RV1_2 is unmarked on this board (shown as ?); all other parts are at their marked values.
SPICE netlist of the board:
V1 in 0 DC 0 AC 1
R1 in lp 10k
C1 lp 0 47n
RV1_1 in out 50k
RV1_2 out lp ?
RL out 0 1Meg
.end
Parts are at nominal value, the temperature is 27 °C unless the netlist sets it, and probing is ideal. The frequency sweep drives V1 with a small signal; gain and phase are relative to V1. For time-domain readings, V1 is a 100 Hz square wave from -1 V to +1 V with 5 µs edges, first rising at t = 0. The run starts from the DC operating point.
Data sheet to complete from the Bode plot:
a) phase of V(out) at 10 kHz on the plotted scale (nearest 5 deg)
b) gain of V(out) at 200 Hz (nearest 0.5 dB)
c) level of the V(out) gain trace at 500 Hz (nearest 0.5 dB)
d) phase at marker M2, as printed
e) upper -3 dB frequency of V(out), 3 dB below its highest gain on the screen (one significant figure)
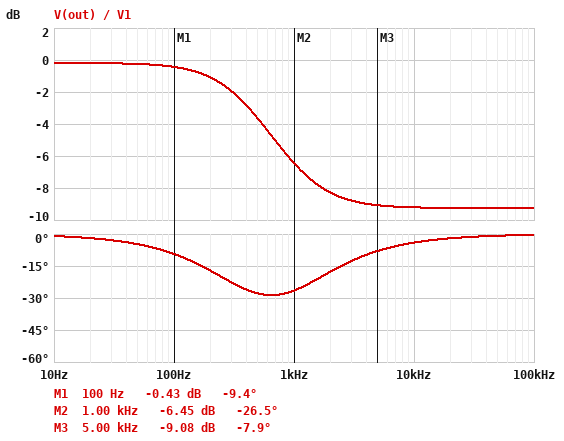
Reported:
-5 deg
-1.0 dB
-3.5 dB
-26.5 deg
400 Hz
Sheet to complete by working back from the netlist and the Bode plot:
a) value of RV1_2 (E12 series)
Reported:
27 kΩ
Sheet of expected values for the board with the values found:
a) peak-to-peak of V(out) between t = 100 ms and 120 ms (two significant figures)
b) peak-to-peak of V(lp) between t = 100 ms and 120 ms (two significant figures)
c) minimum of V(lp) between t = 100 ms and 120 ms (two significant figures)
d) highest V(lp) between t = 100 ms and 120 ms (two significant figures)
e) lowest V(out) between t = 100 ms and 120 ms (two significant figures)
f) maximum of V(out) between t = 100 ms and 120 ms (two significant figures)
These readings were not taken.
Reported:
2.0 V
2.0 V
-990 mV
990 mV
-980 mV
980 mV
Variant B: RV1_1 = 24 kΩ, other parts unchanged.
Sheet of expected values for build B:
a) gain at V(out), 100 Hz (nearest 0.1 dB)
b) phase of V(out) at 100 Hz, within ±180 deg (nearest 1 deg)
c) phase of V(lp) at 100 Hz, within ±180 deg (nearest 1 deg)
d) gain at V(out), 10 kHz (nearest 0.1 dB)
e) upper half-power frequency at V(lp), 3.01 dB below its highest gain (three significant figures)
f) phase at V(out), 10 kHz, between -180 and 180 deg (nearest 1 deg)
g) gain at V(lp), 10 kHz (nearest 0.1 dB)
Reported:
-0.3 dB
-6 deg
-14 deg
-5.6 dB
406 Hz
-2 deg
-27.9 dB
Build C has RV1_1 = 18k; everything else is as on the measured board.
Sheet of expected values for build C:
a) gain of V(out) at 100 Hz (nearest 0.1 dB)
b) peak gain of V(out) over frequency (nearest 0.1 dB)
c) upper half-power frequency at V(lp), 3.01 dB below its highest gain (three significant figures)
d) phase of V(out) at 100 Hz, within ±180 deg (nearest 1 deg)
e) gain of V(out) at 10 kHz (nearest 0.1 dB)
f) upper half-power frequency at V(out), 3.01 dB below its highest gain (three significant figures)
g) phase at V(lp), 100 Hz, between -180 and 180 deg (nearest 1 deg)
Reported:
-0.3 dB
-0.1 dB
414 Hz
-5 deg
-4.5 dB
786 Hz
-14 deg
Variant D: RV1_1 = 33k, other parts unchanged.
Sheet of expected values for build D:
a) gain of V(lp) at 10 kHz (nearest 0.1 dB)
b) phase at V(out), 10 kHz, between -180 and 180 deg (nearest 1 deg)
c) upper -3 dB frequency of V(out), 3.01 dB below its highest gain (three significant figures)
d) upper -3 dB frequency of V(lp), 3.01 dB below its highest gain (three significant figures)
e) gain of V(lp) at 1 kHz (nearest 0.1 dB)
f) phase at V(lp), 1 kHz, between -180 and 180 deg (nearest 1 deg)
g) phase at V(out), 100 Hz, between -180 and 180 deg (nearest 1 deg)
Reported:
-28.1 dB
-3 deg
514 Hz
396 Hz
-8.7 dB
-68 deg
-8 deg
